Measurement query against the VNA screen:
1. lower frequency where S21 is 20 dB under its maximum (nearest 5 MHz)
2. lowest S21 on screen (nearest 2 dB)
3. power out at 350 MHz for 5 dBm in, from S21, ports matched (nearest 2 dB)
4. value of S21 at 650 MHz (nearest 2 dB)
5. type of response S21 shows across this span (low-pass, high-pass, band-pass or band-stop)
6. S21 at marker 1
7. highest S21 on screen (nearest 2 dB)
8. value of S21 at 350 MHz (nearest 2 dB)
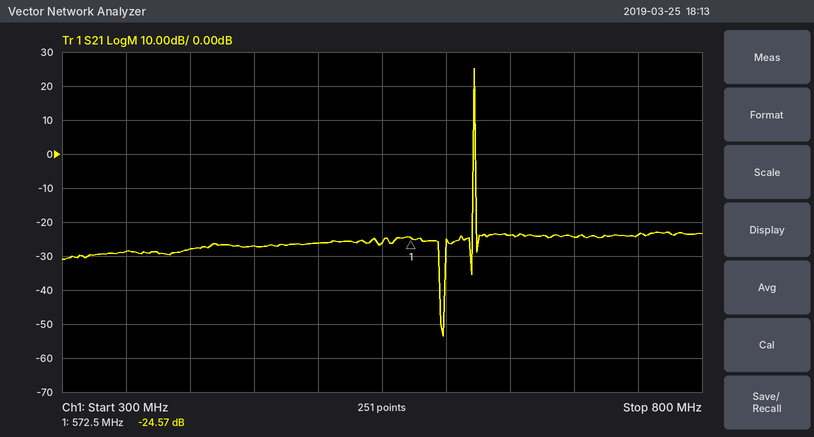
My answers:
620 MHz
-54 dB
-24 dBm
-24 dB
band-pass
-24.57 dB
26 dB
-28 dB
